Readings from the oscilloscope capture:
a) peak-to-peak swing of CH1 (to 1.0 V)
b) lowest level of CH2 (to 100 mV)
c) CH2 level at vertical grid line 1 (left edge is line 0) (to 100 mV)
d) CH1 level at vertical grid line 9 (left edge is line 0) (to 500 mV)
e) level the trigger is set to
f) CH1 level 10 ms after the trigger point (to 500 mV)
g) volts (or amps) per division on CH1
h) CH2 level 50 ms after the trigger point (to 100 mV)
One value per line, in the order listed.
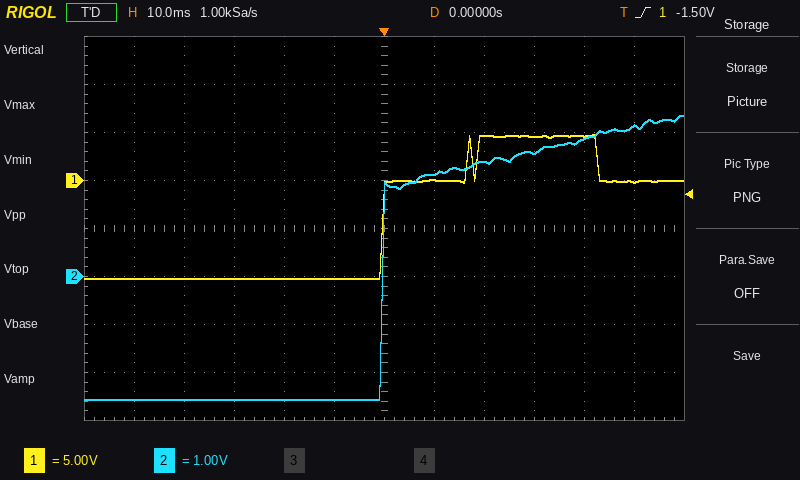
15.0 V
-2.6 V
-2.6 V
4.5 V
-1.50 V
0.0 V
5 V
3.1 V
